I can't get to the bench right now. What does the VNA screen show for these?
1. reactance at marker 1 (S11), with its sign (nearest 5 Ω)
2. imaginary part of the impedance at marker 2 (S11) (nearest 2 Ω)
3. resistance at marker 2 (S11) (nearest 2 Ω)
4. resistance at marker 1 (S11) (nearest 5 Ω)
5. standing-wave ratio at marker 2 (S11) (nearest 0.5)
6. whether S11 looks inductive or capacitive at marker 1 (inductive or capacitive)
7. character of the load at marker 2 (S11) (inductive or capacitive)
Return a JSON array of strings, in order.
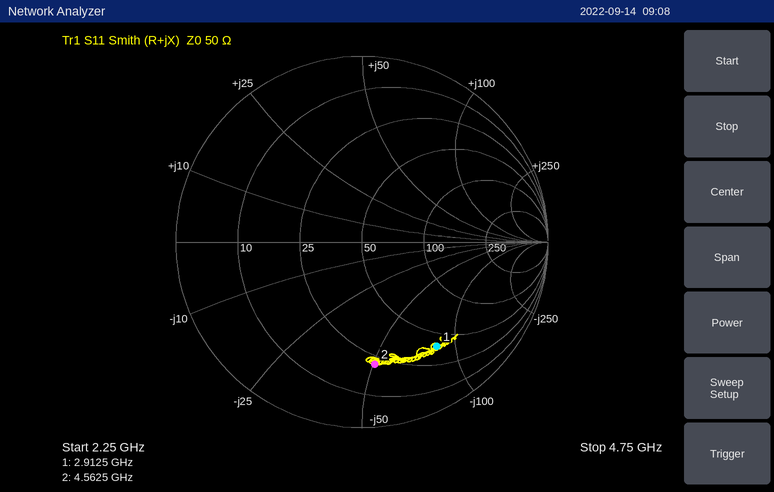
["-85 Ω", "-50 Ω", "22 Ω", "40 Ω", "5.0", "capacitive", "capacitive"]
